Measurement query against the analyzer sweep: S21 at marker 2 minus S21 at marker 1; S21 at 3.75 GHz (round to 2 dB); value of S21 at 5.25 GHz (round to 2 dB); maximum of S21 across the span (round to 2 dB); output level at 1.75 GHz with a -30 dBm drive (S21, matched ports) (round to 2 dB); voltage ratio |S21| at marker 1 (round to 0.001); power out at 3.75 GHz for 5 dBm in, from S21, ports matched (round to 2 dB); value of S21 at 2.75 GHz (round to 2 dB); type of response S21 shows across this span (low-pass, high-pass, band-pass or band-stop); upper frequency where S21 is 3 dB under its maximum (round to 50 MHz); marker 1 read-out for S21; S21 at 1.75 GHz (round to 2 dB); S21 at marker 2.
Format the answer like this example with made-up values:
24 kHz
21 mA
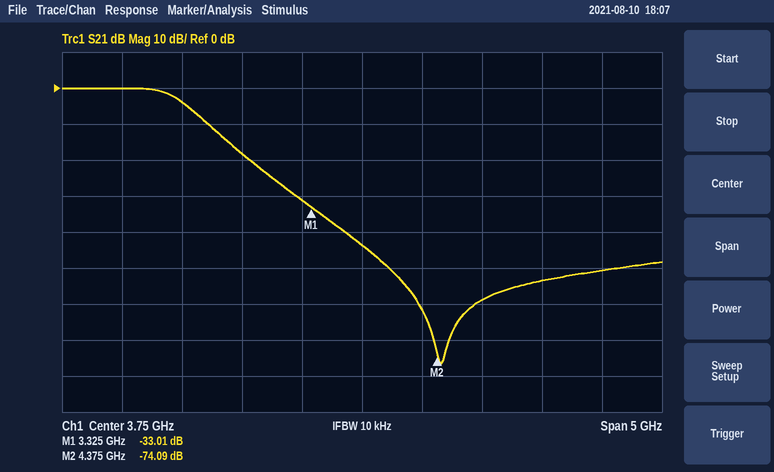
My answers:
-41.08 dB
-44 dB
-54 dB
0 dB
-30 dBm
0.022
-38 dBm
-18 dB
low-pass
2.20 GHz
-33.01 dB
0 dB
-74.09 dB
